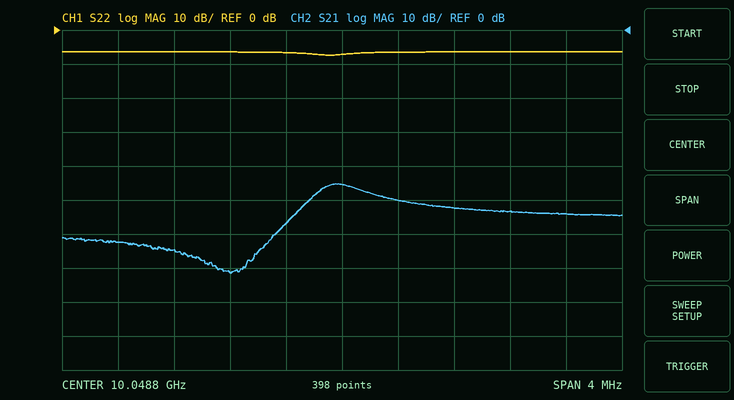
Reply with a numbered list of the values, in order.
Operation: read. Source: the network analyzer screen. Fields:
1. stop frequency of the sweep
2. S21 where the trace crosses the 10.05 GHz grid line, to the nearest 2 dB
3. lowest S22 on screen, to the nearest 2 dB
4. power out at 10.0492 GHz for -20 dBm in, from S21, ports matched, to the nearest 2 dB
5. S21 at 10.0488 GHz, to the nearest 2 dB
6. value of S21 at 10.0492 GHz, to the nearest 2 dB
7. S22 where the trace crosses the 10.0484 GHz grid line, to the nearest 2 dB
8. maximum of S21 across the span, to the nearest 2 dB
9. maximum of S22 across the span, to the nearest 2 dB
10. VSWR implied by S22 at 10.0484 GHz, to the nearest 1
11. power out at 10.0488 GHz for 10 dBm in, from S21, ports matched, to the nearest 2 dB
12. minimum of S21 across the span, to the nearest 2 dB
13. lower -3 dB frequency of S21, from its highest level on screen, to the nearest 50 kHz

1. 10.0508 GHz
2. -54 dB
3. -8 dB
4. -70 dBm
5. -46 dB
6. -50 dB
7. -6 dB
8. -46 dB
9. -6 dB
10. 3
11. -36 dBm
12. -72 dB
13. 10.04860 GHz
